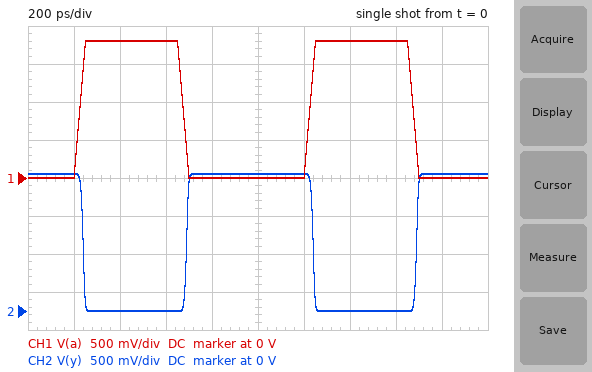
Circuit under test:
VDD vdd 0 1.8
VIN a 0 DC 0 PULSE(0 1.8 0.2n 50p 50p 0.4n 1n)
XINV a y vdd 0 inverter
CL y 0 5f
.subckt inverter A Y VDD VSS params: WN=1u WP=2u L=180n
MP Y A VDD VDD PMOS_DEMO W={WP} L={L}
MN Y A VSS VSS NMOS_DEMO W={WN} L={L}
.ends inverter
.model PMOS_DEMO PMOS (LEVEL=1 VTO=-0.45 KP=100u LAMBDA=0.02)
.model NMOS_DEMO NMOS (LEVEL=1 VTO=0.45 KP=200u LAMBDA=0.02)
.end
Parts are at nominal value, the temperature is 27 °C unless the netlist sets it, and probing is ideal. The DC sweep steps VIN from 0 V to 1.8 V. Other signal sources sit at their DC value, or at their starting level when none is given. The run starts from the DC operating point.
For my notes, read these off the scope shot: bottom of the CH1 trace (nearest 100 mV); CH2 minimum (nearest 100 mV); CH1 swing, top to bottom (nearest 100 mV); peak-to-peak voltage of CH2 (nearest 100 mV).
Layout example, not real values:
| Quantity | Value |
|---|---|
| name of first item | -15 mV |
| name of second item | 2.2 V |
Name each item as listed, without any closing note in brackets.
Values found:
| Quantity | Value |
|---|---|
| bottom of the CH1 trace | 0 V |
| CH2 minimum | 0 V |
| CH1 swing, top to bottom | 1.8 V |
| peak-to-peak voltage of CH2 | 1.8 V |
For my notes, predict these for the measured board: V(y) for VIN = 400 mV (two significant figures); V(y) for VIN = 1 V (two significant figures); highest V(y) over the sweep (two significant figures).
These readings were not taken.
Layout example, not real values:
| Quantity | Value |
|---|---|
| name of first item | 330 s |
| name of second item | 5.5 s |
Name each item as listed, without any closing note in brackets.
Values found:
| Quantity | Value |
|---|---|
| V(y) for VIN = 400 mV | 1.8 V |
| V(y) for VIN = 1 V | 130 mV |
| highest V(y) over the sweep | 1.8 V |
